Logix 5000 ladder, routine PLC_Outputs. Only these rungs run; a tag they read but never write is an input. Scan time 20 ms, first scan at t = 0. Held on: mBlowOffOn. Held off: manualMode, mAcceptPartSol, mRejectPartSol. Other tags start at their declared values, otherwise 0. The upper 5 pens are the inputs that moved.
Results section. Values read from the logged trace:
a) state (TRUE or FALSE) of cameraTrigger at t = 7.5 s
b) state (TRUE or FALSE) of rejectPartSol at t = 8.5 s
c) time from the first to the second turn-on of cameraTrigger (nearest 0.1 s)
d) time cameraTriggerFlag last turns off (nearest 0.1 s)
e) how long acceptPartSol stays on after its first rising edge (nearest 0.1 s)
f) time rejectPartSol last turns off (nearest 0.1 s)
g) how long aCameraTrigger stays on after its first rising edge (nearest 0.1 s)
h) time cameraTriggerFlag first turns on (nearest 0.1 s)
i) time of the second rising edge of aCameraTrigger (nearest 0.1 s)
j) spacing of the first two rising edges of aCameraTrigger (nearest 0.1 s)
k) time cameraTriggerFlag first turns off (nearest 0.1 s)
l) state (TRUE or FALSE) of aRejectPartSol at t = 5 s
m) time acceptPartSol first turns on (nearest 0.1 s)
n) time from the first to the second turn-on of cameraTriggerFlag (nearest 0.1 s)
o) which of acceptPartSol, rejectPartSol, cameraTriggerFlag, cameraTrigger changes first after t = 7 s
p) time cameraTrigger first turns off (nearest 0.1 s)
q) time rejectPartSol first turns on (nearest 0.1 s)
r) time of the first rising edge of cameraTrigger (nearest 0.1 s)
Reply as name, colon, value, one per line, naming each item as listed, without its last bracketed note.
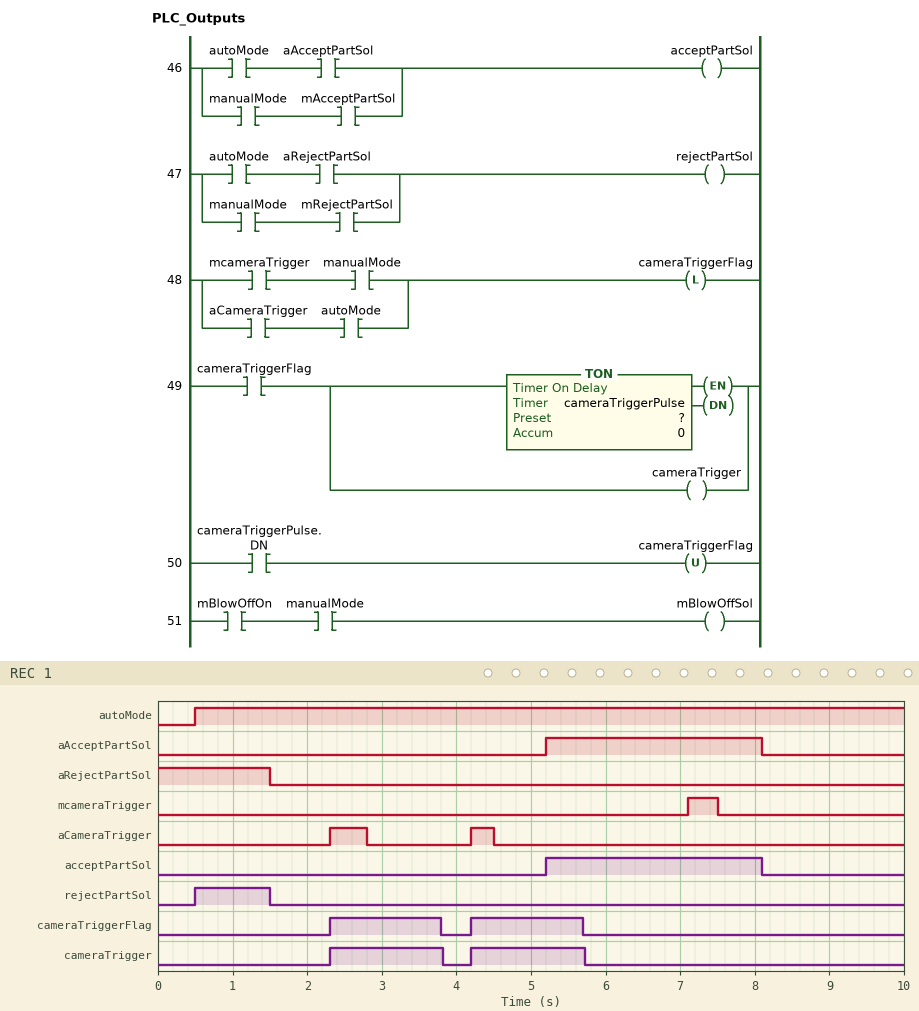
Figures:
state (TRUE or FALSE) of cameraTrigger at t = 7.5 s: FALSE
state (TRUE or FALSE) of rejectPartSol at t = 8.5 s: FALSE
time from the first to the second turn-on of cameraTrigger: 1.9 s
time cameraTriggerFlag last turns off: 5.7 s
how long acceptPartSol stays on after its first rising edge: 2.9 s
time rejectPartSol last turns off: 1.5 s
how long aCameraTrigger stays on after its first rising edge: 0.5 s
time cameraTriggerFlag first turns on: 2.3 s
time of the second rising edge of aCameraTrigger: 4.2 s
spacing of the first two rising edges of aCameraTrigger: 1.9 s
time cameraTriggerFlag first turns off: 3.8 s
state (TRUE or FALSE) of aRejectPartSol at t = 5 s: FALSE
time acceptPartSol first turns on: 5.2 s
time from the first to the second turn-on of cameraTriggerFlag: 1.9 s
which of acceptPartSol, rejectPartSol, cameraTriggerFlag, cameraTrigger changes first after t = 7 s: acceptPartSol
time cameraTrigger first turns off: 3.8 s
time rejectPartSol first turns on: 0.5 s
time of the first rising edge of cameraTrigger: 2.3 s
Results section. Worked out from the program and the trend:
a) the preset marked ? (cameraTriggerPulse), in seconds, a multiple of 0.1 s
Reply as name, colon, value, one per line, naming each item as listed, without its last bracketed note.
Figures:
the preset marked ? (cameraTriggerPulse), in seconds, a multiple of 0.1 s: 1.5 s
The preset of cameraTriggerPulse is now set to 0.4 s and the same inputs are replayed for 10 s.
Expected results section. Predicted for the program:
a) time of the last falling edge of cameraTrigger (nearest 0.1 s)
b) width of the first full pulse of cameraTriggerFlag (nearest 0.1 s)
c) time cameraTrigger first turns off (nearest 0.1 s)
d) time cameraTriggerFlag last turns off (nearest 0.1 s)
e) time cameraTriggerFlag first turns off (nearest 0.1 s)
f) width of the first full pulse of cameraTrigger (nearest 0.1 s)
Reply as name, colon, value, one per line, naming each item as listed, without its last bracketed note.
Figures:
time of the last falling edge of cameraTrigger: 4.6 s
width of the first full pulse of cameraTriggerFlag: 0.4 s
time cameraTrigger first turns off: 2.8 s
time cameraTriggerFlag last turns off: 4.6 s
time cameraTriggerFlag first turns off: 2.7 s
width of the first full pulse of cameraTrigger: 0.5 s
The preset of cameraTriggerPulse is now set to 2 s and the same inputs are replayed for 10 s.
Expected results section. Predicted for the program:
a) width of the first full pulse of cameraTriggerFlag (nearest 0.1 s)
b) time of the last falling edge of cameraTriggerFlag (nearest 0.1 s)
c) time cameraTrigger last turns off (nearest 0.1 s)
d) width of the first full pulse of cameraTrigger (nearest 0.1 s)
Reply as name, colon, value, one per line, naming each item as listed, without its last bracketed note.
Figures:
width of the first full pulse of cameraTriggerFlag: 2.0 s
time of the last falling edge of cameraTriggerFlag: 4.3 s
time cameraTrigger last turns off: 4.5 s
width of the first full pulse of cameraTrigger: 2.2 s
